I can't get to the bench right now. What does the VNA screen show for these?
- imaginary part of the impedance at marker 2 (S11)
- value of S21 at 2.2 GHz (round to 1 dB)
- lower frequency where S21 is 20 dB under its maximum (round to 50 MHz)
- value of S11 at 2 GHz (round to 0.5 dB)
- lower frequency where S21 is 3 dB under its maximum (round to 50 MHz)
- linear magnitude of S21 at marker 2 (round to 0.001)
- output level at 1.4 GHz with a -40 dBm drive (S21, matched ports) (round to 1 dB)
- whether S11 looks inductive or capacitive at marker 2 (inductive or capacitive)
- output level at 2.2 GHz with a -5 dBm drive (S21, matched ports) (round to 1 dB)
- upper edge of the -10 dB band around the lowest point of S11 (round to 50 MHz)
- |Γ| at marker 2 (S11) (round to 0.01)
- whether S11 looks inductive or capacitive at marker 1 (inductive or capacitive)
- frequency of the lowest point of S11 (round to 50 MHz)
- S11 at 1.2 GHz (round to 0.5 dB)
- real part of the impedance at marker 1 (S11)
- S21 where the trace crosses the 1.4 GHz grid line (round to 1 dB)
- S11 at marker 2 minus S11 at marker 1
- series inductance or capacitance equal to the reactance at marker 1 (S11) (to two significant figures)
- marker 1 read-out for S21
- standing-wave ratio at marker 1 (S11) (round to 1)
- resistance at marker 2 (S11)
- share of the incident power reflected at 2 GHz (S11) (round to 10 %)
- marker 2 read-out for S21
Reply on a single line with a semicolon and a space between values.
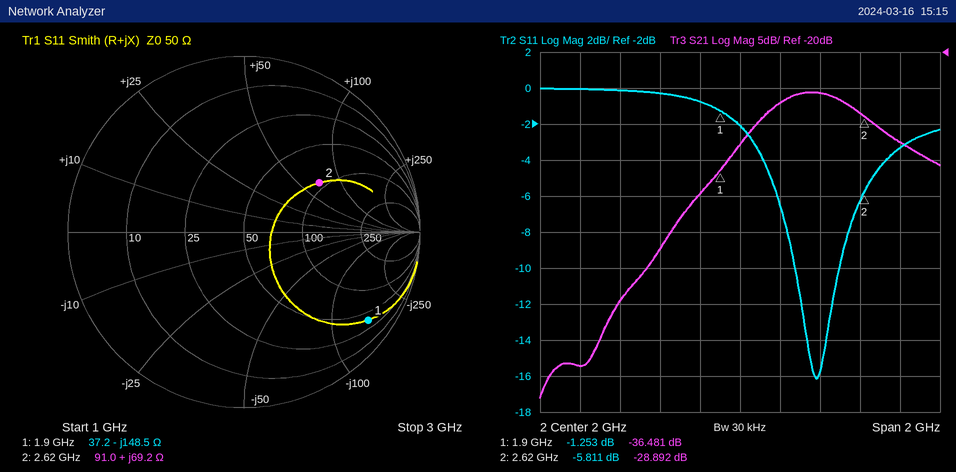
+69.2 Ω; -27 dB; 1.65 GHz; -2.0 dB; 2.15 GHz; 0.036; -95 dBm; inductive; -32 dBm; 2.50 GHz; 0.51; capacitive; 2.40 GHz; 0.0 dB; 37.2 Ω; -55 dB; -4.558 dB; 560 fF; -36.481 dB; 14; 91.0 Ω; 60 %; -28.892 dB
